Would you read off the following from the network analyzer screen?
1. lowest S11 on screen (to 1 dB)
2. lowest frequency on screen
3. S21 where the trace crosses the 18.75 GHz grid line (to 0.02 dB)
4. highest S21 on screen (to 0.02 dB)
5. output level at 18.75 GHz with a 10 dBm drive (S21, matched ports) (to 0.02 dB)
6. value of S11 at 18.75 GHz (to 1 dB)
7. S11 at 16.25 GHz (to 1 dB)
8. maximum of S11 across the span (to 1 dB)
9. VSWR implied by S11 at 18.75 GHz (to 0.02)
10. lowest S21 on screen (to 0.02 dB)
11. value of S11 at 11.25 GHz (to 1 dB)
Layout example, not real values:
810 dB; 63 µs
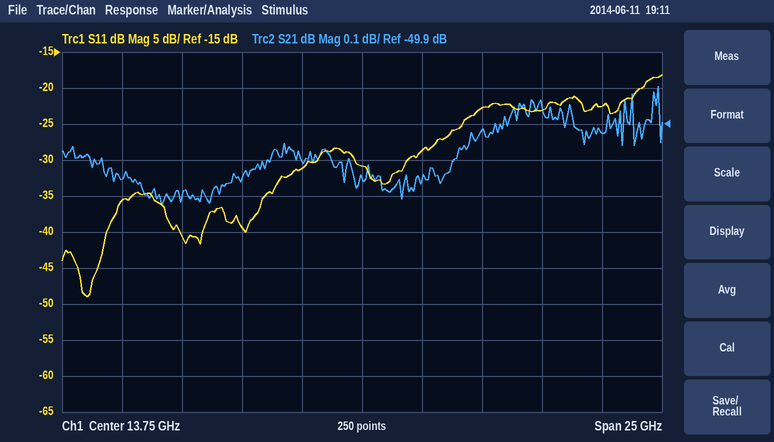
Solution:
-49 dB; 1.25 GHz; -49.92 dB; -49.80 dB; -39.92 dBm; -23 dB; -29 dB; -18 dB; 1.16; -50.12 dB; -31 dB
